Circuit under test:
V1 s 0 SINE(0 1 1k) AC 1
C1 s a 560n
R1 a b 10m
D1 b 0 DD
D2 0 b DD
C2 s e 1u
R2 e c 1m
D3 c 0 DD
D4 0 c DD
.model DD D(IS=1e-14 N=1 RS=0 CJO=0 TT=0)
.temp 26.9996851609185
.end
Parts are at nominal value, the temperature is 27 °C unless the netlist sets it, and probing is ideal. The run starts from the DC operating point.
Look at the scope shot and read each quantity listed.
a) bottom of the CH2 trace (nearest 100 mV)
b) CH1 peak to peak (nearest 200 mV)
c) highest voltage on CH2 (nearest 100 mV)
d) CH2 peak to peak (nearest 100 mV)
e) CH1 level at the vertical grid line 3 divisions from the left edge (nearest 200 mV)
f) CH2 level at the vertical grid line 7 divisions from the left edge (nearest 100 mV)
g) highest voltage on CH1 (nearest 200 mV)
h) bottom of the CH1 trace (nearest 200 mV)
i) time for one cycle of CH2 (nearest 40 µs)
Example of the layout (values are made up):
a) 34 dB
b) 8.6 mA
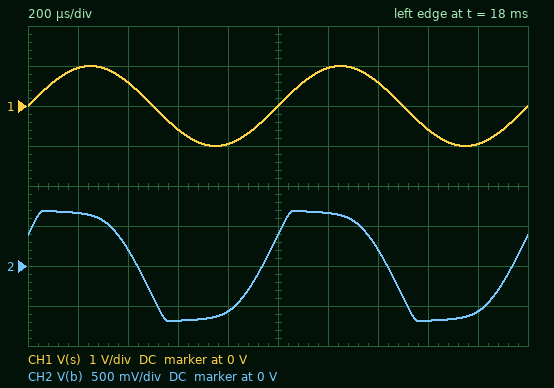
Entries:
a) -700 mV
b) 2.0 V
c) 700 mV
d) 1.4 V
e) -600 mV
f) 200 mV
g) 1.0 V
h) -1.0 V
i) 1.00 ms
